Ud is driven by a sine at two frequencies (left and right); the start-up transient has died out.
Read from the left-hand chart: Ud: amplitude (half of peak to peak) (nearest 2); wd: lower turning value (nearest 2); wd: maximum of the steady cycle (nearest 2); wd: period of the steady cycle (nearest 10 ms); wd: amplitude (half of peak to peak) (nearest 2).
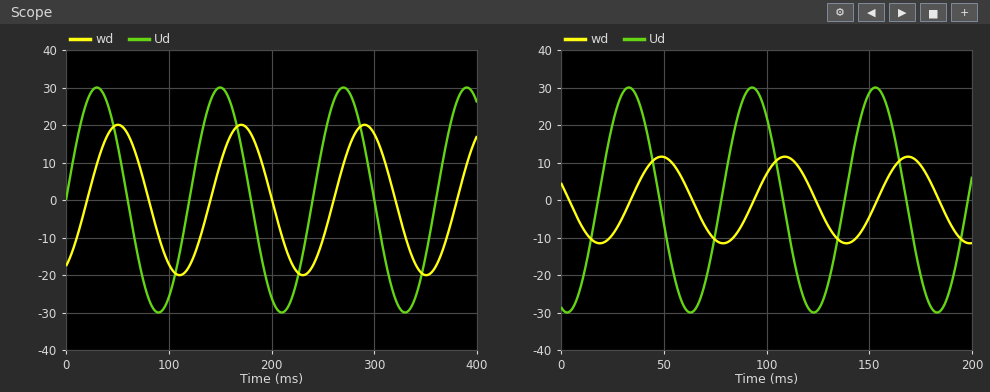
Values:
30
-20
20
120 ms
20
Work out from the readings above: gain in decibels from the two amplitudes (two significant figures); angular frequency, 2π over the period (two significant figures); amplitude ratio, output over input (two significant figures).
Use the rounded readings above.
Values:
-3.5 dB
0.052 rad/ms
0.67
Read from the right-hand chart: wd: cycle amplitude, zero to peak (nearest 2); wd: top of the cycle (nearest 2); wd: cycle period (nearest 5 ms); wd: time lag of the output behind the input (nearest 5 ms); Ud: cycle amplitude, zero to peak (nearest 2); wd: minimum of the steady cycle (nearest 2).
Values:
12
12
60 ms
15 ms
30
-12
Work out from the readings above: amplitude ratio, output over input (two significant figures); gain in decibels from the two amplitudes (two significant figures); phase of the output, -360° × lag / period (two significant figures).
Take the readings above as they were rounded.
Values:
0.40
-8.0 dB
-90°
